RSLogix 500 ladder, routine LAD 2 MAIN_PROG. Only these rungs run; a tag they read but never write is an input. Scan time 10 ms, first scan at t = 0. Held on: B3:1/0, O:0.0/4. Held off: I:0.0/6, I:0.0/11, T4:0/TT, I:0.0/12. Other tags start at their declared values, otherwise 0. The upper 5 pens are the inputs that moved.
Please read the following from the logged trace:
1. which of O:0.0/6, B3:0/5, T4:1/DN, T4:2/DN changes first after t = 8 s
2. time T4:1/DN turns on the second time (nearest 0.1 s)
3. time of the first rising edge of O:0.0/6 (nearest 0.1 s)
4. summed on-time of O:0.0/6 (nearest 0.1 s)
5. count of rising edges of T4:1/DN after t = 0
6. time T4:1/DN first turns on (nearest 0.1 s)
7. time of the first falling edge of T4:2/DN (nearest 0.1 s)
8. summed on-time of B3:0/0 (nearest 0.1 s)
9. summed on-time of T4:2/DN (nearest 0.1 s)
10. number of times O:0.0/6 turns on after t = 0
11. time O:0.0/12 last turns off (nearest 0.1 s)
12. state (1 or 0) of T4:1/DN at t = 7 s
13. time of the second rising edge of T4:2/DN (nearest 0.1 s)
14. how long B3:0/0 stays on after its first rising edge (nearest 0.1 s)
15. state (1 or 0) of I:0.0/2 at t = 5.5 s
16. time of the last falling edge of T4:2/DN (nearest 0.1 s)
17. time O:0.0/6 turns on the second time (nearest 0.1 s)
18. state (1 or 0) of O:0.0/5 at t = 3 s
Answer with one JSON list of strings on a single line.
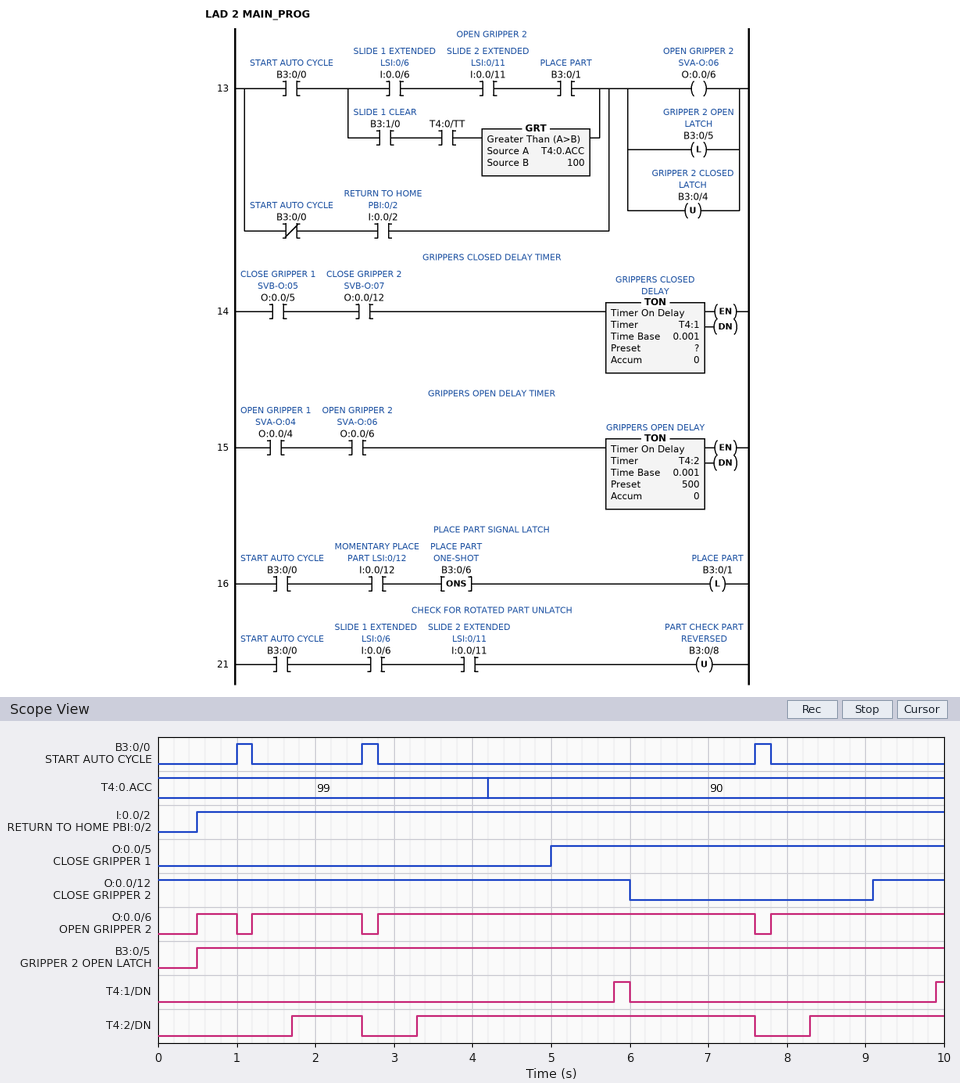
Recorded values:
["T4:2/DN", "9.9 s", "0.5 s", "8.9 s", "2", "5.8 s", "2.6 s", "0.6 s", "6.9 s", "4", "6.0 s", "0", "3.3 s", "0.2 s", "1", "7.6 s", "1.2 s", "0"]
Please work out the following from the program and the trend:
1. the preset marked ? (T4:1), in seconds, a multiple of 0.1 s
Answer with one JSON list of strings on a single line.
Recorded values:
["0.8 s"]
